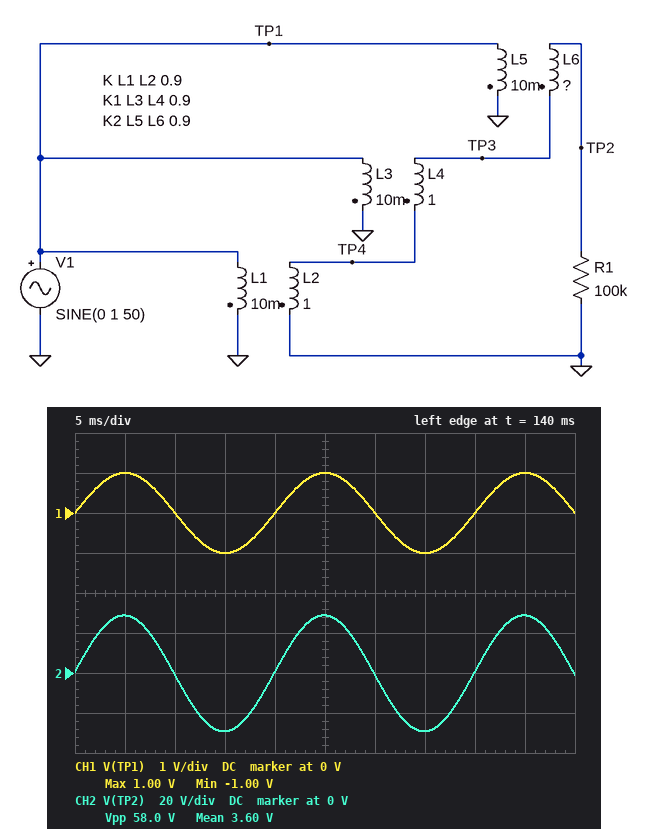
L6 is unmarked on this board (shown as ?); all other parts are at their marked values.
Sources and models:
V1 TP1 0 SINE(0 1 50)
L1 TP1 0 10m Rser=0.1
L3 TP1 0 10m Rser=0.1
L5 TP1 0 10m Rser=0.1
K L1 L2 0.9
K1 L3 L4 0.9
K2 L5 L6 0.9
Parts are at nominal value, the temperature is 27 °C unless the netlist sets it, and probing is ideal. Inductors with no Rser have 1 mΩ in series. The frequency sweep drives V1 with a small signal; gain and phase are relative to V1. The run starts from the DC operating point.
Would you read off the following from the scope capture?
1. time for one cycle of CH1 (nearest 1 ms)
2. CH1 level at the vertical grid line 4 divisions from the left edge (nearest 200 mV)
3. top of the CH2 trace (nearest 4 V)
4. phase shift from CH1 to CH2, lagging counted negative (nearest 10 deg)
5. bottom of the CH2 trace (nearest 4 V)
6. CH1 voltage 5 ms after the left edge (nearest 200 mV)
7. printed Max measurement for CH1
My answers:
20 ms
0 V
28 V
0 deg
-28 V
1.0 V
1.00 V
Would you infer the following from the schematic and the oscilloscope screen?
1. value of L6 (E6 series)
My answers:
1.5 H
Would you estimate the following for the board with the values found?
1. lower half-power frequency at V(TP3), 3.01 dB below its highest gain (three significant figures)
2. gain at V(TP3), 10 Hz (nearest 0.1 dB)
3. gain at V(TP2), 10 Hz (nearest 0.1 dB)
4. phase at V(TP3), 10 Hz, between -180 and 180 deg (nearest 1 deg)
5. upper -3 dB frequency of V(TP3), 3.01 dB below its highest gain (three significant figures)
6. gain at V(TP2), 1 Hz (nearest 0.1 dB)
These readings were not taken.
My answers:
1.59 Hz
25.0 dB
29.1 dB
9 deg
24.1 kHz
23.8 dB
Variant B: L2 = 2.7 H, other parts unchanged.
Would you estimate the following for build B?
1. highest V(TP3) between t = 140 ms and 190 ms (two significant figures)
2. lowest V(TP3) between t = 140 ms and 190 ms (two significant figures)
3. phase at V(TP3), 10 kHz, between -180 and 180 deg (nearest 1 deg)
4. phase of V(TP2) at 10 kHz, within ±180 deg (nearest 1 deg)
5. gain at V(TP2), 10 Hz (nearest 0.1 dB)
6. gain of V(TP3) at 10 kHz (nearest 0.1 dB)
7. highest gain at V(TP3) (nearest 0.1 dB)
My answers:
24 V
-24 V
-33 deg
-32 deg
30.7 dB
26.1 dB
27.5 dB
